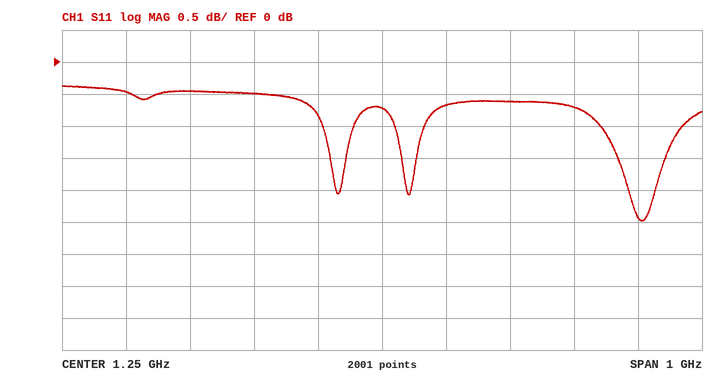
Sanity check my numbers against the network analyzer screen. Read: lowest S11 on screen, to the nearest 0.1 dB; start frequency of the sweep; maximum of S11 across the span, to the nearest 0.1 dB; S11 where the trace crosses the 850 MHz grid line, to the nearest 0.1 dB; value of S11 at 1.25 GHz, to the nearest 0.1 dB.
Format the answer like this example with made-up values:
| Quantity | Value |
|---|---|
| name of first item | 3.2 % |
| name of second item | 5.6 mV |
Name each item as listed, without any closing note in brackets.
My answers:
| Quantity | Value |
|---|---|
| lowest S11 on screen, to the nearest 0.1 dB | -2.5 dB |
| start frequency of the sweep | 750 MHz |
| maximum of S11 across the span, to the nearest 0.1 dB | -0.4 dB |
| S11 where the trace crosses the 850 MHz grid line, to the nearest 0.1 dB | -0.5 dB |
| value of S11 at 1.25 GHz, to the nearest 0.1 dB | -0.7 dB |
